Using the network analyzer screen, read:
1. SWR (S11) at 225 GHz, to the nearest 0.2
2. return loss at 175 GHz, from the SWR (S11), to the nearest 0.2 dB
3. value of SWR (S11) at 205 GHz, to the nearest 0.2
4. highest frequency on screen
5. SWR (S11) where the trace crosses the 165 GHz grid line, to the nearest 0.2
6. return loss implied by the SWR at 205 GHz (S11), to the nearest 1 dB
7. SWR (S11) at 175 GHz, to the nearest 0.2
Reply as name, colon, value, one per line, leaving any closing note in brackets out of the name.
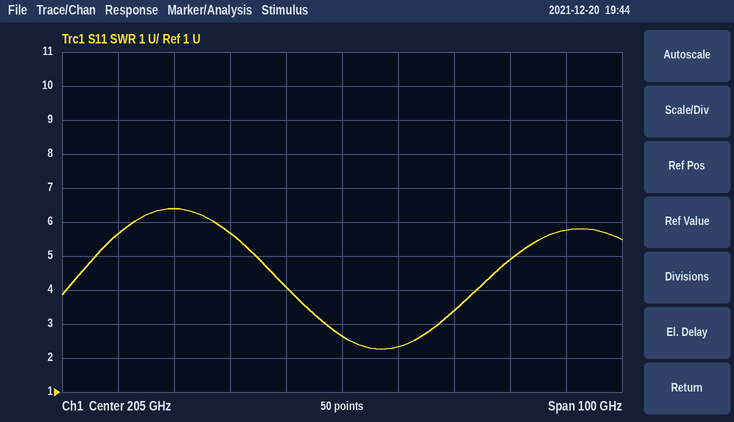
SWR (S11) at 225 GHz, to the nearest 0.2: 3.4
return loss at 175 GHz, from the SWR (S11), to the nearest 0.2 dB: 2.8 dB
value of SWR (S11) at 205 GHz, to the nearest 0.2: 2.6
highest frequency on screen: 255 GHz
SWR (S11) where the trace crosses the 165 GHz grid line, to the nearest 0.2: 5.6
return loss implied by the SWR at 205 GHz (S11), to the nearest 1 dB: 7 dB
SWR (S11) at 175 GHz, to the nearest 0.2: 6.4
